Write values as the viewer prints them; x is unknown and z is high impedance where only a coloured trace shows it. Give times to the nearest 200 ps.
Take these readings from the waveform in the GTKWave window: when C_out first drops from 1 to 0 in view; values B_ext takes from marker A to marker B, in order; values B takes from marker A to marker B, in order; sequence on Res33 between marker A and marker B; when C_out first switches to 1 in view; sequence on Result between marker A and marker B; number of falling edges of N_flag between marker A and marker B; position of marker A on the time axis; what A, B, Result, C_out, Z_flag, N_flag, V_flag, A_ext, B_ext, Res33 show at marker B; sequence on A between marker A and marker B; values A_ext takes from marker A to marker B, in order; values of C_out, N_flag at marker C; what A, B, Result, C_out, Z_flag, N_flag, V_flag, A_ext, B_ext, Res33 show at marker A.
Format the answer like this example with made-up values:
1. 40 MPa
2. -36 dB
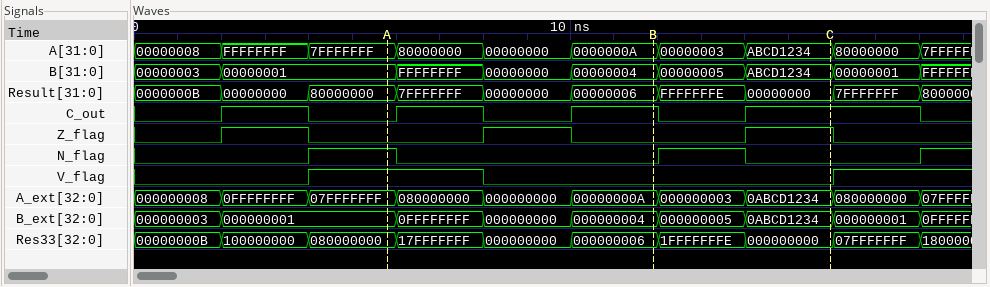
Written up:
1. 4000 ps
2. 000000001, 0FFFFFFFF, 000000000, 000000004
3. 00000001, FFFFFFFF, 00000000, 00000004
4. 080000000, 17FFFFFFF, 000000000, 000000006
5. 2000 ps
6. 80000000, 7FFFFFFF, 00000000, 00000006
7. 1
8. 5800 ps
9. A=0000000A, B=00000004, Result=00000006, C_out=1, Z_flag=0, N_flag=0, V_flag=0, A_ext=00000000A, B_ext=000000004, Res33=000000006
10. 7FFFFFFF, 80000000, 00000000, 0000000A
11. 07FFFFFFF, 080000000, 000000000, 00000000A
12. C_out=1, N_flag=0
13. A=7FFFFFFF, B=00000001, Result=80000000, C_out=0, Z_flag=0, N_flag=1, V_flag=1, A_ext=07FFFFFFF, B_ext=000000001, Res33=080000000
